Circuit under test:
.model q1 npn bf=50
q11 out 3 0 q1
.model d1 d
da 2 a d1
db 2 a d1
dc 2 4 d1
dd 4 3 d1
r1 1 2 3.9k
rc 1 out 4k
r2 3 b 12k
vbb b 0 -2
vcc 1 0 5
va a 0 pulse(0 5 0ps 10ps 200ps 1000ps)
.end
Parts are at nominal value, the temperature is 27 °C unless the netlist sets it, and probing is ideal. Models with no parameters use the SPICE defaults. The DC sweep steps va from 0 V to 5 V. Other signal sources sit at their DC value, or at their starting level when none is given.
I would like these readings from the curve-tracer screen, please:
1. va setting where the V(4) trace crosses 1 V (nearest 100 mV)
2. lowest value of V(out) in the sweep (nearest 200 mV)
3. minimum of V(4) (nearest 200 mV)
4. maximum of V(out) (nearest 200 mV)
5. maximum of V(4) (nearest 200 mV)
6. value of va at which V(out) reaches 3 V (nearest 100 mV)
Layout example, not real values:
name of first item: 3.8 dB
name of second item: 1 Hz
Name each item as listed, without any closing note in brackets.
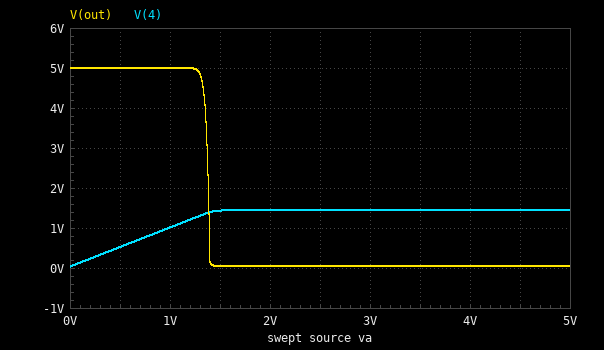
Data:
va setting where the V(4) trace crosses 1 V: 1.0 V
lowest value of V(out) in the sweep: 0 V
minimum of V(4): 0 V
maximum of V(out): 5.0 V
maximum of V(4): 1.4 V
value of va at which V(out) reaches 3 V: 1.4 V
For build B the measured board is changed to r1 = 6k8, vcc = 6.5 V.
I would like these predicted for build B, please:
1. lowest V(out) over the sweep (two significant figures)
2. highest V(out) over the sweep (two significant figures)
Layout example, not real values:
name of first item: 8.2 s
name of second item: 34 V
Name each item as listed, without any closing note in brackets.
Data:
lowest V(out) over the sweep: 48 mV
highest V(out) over the sweep: 6.5 V
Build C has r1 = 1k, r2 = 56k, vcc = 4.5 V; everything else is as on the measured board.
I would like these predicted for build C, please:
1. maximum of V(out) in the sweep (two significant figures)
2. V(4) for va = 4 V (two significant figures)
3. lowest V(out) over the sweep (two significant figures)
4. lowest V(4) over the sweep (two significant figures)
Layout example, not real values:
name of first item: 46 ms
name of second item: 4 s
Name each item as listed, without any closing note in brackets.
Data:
maximum of V(out) in the sweep: 4.5 V
V(4) for va = 4 V: 1.5 V
lowest V(out) over the sweep: 24 mV
lowest V(4) over the sweep: 110 mV
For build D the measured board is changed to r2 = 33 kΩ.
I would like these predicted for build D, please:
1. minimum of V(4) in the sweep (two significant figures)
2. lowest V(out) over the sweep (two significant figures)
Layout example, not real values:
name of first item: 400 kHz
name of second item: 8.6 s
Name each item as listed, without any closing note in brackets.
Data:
minimum of V(4) in the sweep: 64 mV
lowest V(out) over the sweep: 36 mV
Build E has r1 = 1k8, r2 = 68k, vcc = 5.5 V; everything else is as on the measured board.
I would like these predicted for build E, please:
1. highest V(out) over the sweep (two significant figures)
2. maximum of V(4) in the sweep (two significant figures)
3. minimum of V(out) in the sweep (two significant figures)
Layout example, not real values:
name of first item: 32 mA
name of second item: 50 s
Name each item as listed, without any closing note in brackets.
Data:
highest V(out) over the sweep: 5.5 V
maximum of V(4) in the sweep: 1.5 V
minimum of V(out) in the sweep: 27 mV
